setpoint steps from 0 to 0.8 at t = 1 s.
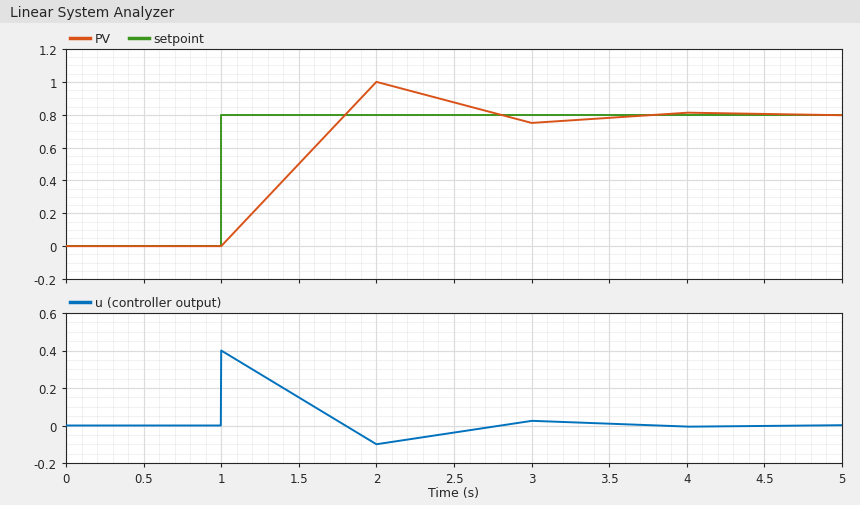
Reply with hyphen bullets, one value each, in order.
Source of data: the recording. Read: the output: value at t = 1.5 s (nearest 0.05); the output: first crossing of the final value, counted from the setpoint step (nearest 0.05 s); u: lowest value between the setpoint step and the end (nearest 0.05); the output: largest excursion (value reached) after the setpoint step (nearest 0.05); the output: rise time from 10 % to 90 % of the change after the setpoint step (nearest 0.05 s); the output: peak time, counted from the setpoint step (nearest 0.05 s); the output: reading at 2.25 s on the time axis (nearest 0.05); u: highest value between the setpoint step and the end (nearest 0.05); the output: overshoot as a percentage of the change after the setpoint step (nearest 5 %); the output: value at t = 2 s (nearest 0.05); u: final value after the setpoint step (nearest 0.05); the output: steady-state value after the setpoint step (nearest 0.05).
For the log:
- 0.50
- 0.80 s
- -0.10
- 1.00
- 0.65 s
- 1.00 s
- 0.95
- 0.40
- 25 %
- 1.00
- 0.00
- 0.80
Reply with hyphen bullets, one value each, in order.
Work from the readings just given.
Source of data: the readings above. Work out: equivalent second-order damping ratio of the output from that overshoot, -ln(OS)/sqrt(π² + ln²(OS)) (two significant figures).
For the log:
- 0.40
